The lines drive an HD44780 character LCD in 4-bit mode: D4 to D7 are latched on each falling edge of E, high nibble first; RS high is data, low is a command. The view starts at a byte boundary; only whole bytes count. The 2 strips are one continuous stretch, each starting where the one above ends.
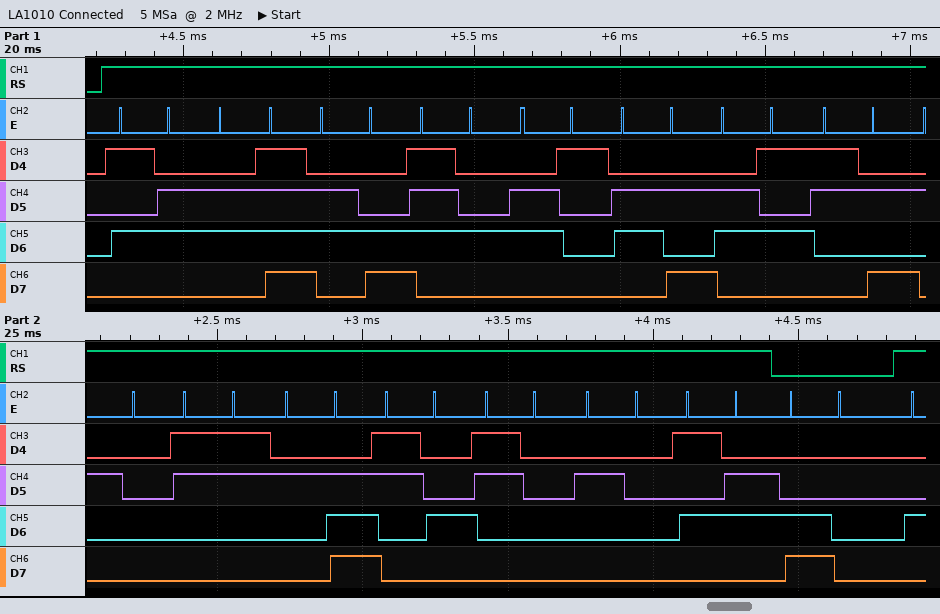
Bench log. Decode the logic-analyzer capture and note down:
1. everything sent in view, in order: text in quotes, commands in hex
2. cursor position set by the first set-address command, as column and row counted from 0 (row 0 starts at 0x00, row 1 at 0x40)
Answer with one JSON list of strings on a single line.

["\"Voltaje: 3.40 V\" 0xC0", "column 0, row 1"]
